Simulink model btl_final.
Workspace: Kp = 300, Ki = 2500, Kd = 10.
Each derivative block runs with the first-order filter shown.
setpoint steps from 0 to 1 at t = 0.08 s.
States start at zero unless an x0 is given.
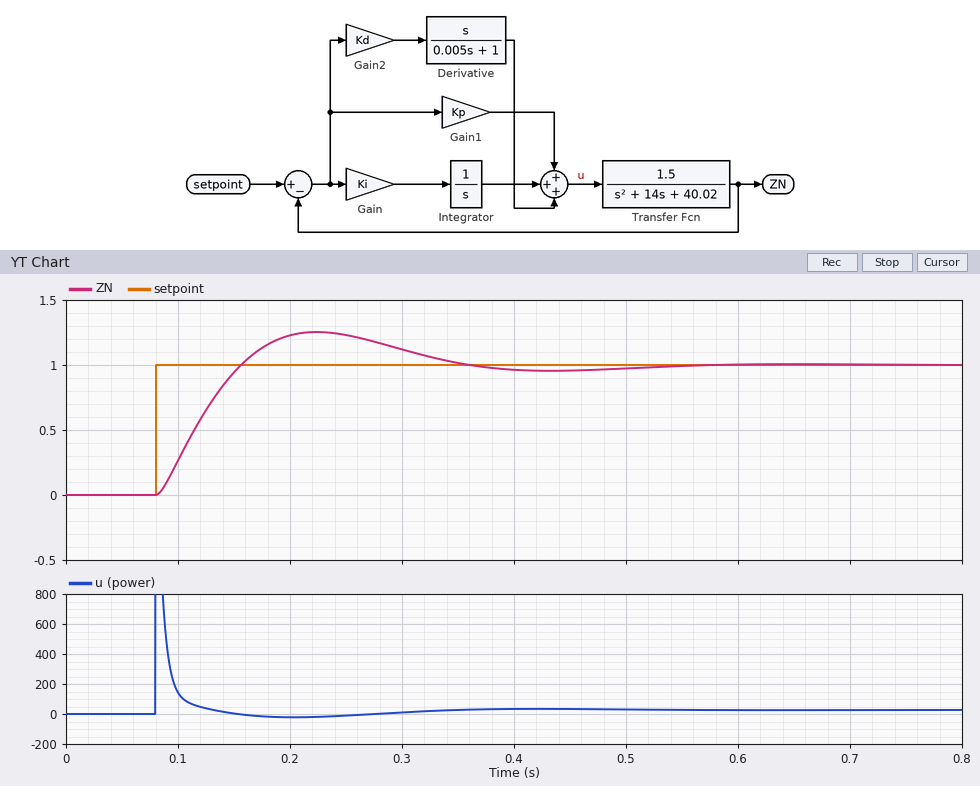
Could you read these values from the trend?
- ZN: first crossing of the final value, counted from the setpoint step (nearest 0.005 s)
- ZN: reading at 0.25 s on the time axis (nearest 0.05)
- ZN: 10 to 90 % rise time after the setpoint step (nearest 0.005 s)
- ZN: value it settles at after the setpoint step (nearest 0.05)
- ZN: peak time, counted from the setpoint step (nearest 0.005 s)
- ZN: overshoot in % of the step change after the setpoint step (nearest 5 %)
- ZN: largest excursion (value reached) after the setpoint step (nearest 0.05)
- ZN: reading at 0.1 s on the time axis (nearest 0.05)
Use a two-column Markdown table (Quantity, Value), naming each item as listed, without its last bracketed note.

| Quantity | Value |
|---|---|
| ZN: first crossing of the final value, counted from the setpoint step | 0.075 s |
| ZN: reading at 0.25 s on the time axis | 1.25 |
| ZN: 10 to 90 % rise time after the setpoint step | 0.055 s |
| ZN: value it settles at after the setpoint step | 1.00 |
| ZN: peak time, counted from the setpoint step | 0.145 s |
| ZN: overshoot in % of the step change after the setpoint step | 25 % |
| ZN: largest excursion (value reached) after the setpoint step | 1.25 |
| ZN: reading at 0.1 s on the time axis | 0.25 |
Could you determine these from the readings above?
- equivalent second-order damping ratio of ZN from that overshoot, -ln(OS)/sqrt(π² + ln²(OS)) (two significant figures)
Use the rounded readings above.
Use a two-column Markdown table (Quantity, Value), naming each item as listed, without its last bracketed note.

| Quantity | Value |
|---|---|
| equivalent second-order damping ratio of ZN from that overshoot, -ln(OS)/sqrt(π² + ln²(OS)) | 0.40 |
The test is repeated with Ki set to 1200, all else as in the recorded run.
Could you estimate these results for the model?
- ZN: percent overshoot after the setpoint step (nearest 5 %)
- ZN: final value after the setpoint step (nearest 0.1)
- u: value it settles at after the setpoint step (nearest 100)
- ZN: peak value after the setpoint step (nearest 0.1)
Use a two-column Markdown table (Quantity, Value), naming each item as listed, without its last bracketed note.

| Quantity | Value |
|---|---|
| ZN: percent overshoot after the setpoint step | 15 % |
| ZN: final value after the setpoint step | 1.0 |
| u: value it settles at after the setpoint step | 0 |
| ZN: peak value after the setpoint step | 1.1 |
